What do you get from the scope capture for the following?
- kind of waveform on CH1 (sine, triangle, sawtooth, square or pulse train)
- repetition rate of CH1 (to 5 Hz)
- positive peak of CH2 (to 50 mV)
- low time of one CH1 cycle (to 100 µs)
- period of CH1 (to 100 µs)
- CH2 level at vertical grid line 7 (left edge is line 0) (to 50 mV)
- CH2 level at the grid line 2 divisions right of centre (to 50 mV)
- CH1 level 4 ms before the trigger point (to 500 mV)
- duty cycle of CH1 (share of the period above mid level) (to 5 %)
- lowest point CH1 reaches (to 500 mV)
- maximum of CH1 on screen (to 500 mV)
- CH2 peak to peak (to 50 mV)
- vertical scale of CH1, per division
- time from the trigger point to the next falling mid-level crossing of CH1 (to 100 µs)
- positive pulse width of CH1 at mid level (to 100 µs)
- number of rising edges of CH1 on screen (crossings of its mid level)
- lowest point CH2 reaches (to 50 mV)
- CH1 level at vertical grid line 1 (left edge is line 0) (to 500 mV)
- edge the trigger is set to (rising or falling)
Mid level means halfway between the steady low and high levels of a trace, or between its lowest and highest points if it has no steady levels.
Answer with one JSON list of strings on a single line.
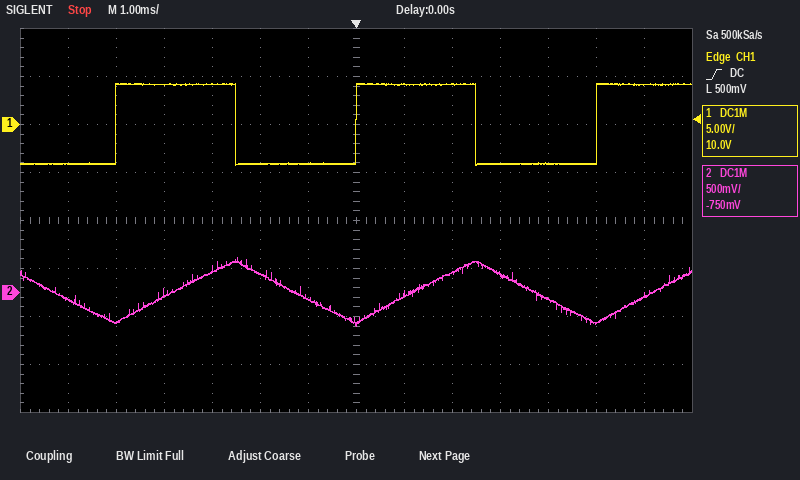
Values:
["square", "200 Hz", "350 mV", "2.5 ms", "5.0 ms", "-300 mV", "200 mV", "4.0 V", "50 %", "-4.5 V", "4.5 V", "700 mV", "5 V", "2.5 ms", "2.5 ms", "3", "-350 mV", "-4.0 V", "rising"]
